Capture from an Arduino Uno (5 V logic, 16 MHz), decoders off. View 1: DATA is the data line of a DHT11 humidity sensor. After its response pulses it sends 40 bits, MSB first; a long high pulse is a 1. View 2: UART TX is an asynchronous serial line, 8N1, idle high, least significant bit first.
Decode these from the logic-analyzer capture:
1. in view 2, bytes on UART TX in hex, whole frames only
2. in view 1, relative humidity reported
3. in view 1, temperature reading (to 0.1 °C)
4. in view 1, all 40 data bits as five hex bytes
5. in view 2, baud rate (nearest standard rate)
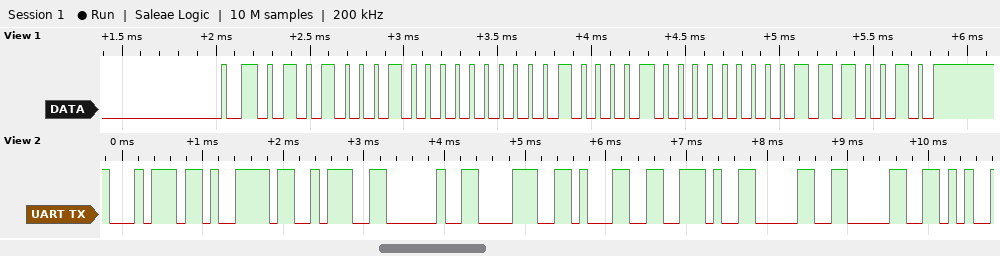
74 79 3A 20 38 31 2E 30 30
81 %
33.0 °C
51 00 21 00 72
9600 baud
